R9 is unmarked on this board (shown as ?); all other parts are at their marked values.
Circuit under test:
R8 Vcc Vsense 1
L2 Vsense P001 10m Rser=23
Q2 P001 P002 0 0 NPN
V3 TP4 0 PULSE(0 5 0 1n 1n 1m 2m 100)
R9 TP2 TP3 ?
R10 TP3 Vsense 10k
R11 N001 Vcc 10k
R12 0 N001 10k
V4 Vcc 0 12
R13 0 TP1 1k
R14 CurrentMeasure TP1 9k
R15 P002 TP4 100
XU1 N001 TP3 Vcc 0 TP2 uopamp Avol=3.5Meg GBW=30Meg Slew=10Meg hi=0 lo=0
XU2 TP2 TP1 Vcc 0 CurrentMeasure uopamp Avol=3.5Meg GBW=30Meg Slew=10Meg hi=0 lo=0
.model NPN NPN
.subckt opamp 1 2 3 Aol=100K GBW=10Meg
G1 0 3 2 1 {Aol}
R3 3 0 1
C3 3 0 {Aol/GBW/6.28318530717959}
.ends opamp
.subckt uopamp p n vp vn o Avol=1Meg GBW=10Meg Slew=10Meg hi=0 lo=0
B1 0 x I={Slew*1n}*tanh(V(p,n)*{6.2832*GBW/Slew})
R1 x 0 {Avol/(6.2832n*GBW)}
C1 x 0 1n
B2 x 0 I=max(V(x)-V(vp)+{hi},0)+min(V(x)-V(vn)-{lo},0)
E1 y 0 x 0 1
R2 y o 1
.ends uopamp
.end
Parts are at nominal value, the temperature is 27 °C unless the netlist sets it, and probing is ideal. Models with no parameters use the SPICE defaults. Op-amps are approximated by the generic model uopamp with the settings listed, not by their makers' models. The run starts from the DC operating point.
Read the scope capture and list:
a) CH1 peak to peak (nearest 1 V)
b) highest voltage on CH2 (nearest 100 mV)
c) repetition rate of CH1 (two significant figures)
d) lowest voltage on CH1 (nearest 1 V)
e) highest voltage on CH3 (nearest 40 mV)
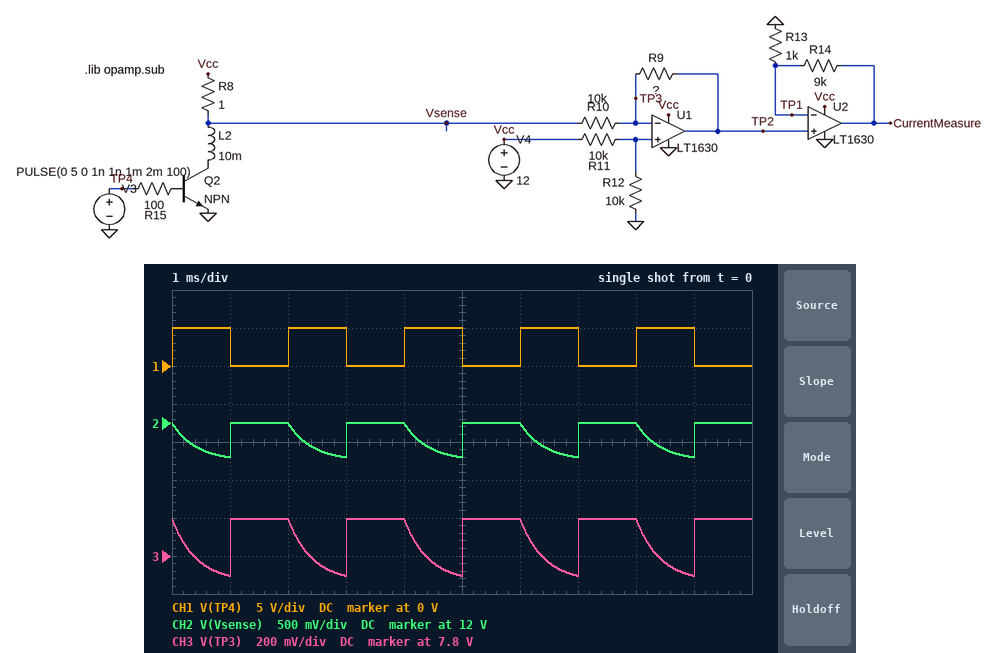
5 V
12.0 V
500 Hz
0 V
8.00 V
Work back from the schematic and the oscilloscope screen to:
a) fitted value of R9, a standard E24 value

20 kΩ
